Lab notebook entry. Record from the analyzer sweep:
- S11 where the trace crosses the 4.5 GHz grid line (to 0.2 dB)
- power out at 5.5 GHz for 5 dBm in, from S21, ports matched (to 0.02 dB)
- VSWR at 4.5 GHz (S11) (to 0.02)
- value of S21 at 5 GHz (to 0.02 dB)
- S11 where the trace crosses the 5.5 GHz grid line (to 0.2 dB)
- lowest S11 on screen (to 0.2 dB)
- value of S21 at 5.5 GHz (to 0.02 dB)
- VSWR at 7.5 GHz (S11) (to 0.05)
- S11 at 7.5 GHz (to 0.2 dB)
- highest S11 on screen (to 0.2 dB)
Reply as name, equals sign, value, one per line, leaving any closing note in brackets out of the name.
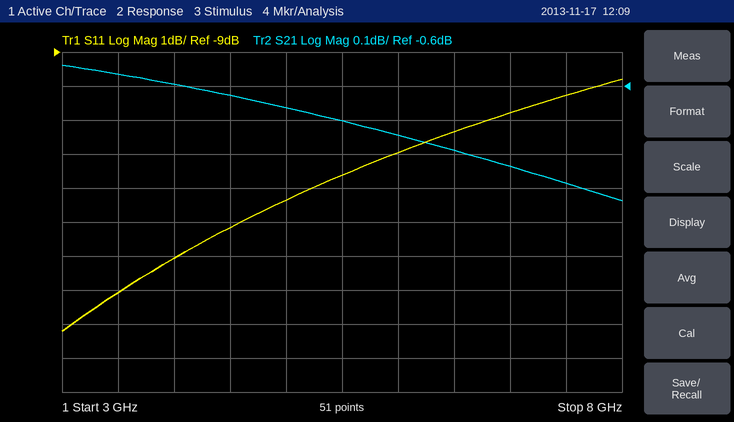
S11 where the trace crosses the 4.5 GHz grid line = -14.2 dB
power out at 5.5 GHz for 5 dBm in, from S21, ports matched = 4.30 dBm
VSWR at 4.5 GHz (S11) = 1.48
value of S21 at 5 GHz = -0.66 dB
S11 where the trace crosses the 5.5 GHz grid line = -12.6 dB
lowest S11 on screen = -17.2 dB
value of S21 at 5.5 GHz = -0.70 dB
VSWR at 7.5 GHz (S11) = 1.90
S11 at 7.5 GHz = -10.2 dB
highest S11 on screen = -9.8 dB
